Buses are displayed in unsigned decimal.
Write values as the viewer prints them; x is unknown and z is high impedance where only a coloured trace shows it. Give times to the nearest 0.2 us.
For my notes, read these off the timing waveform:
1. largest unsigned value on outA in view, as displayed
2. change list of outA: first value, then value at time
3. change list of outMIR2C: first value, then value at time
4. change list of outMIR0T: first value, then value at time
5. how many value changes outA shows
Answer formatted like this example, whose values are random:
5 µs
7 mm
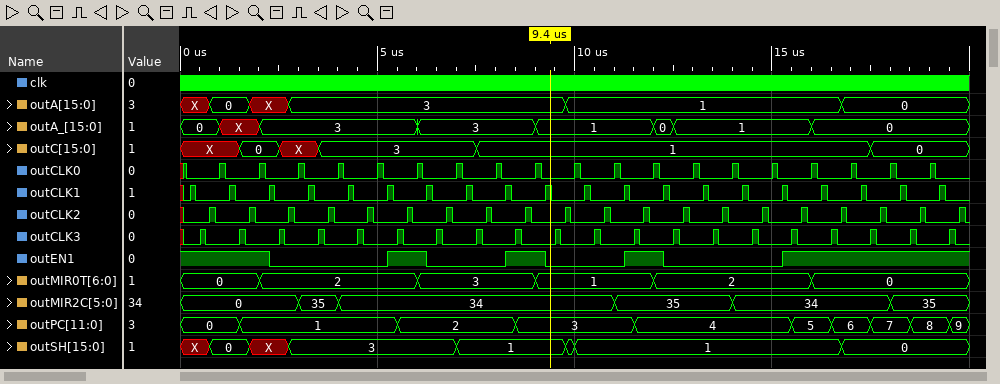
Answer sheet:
3
X, 0 at 0.8 us, X at 1.8 us, 3 at 2.8 us, 1 at 9.8 us, 0 at 16.8 us
0, 35 at 3 us, 34 at 4 us, 35 at 11 us, 34 at 14 us, 35 at 18 us
0, 2 at 2 us, 3 at 6 us, 1 at 9 us, 2 at 12 us, 0 at 16 us
5
